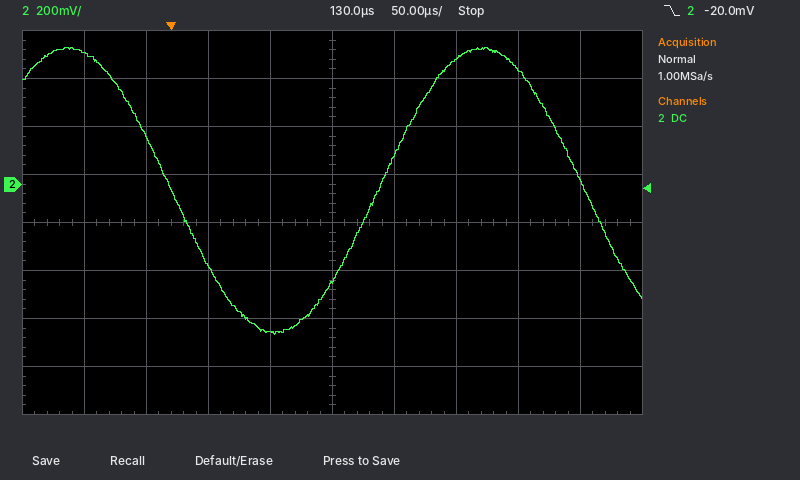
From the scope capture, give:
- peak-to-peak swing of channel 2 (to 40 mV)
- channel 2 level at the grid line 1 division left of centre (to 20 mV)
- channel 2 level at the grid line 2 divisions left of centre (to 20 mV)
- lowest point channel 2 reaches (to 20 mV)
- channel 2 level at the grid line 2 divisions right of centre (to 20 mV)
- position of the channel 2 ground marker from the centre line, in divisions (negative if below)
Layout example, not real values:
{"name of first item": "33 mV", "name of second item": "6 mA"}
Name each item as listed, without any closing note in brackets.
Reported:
{"peak-to-peak swing of channel 2": "1.20 V", "channel 2 level at the grid line 1 division left of centre": "-620 mV", "channel 2 level at the grid line 2 divisions left of centre": "-340 mV", "lowest point channel 2 reaches": "-620 mV", "channel 2 level at the grid line 2 divisions right of centre": "520 mV", "position of the channel 2 ground marker from the centre line, in divisions": "+0.8 div"}
